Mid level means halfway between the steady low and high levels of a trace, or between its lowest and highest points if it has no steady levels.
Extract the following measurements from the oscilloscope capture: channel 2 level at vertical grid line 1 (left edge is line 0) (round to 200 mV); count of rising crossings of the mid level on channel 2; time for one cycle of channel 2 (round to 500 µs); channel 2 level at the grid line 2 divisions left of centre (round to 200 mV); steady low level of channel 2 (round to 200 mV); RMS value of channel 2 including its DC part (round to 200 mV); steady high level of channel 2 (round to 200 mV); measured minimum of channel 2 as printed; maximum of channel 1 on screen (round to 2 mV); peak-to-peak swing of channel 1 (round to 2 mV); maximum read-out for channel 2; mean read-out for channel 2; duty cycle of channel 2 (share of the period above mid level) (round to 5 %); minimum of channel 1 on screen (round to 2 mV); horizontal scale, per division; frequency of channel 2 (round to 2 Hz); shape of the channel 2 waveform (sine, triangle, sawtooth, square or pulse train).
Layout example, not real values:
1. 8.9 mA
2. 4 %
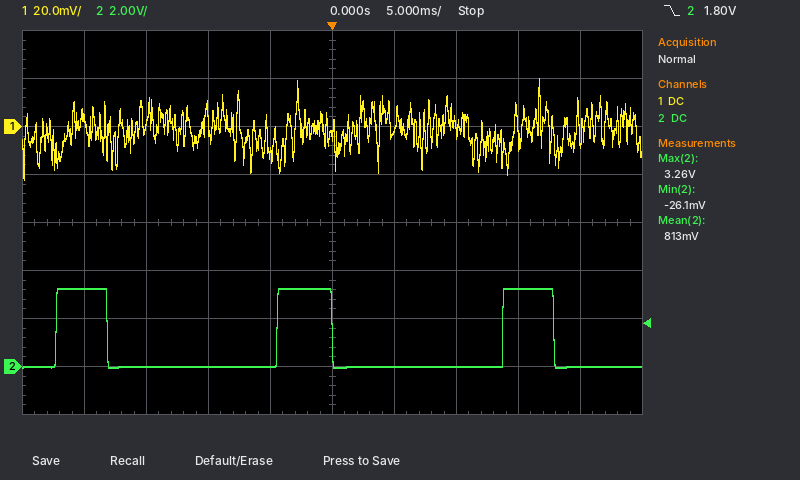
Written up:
1. 3.2 V
2. 3
3. 18.0 ms
4. 0.0 V
5. 0.0 V
6. 1.6 V
7. 3.2 V
8. -26.1 mV
9. 20 mV
10. 42 mV
11. 3.26 V
12. 813 mV
13. 25 %
14. -22 mV
15. 5 ms
16. 56 Hz
17. pulse train
